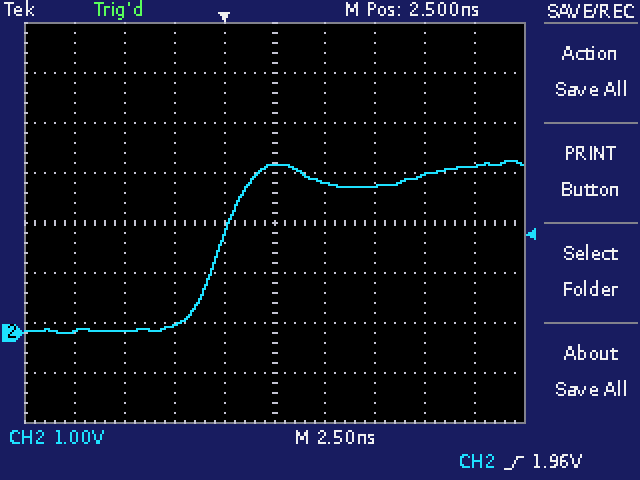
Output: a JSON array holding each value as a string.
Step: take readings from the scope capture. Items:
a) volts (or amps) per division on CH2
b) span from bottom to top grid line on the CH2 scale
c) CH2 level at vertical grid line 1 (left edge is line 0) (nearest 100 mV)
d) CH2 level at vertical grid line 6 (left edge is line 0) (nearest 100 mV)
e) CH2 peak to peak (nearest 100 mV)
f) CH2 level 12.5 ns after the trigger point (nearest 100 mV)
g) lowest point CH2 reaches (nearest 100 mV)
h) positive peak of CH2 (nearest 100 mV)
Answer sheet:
["1 V", "8 V", "0.0 V", "3.0 V", "3.4 V", "3.3 V", "0.0 V", "3.4 V"]
